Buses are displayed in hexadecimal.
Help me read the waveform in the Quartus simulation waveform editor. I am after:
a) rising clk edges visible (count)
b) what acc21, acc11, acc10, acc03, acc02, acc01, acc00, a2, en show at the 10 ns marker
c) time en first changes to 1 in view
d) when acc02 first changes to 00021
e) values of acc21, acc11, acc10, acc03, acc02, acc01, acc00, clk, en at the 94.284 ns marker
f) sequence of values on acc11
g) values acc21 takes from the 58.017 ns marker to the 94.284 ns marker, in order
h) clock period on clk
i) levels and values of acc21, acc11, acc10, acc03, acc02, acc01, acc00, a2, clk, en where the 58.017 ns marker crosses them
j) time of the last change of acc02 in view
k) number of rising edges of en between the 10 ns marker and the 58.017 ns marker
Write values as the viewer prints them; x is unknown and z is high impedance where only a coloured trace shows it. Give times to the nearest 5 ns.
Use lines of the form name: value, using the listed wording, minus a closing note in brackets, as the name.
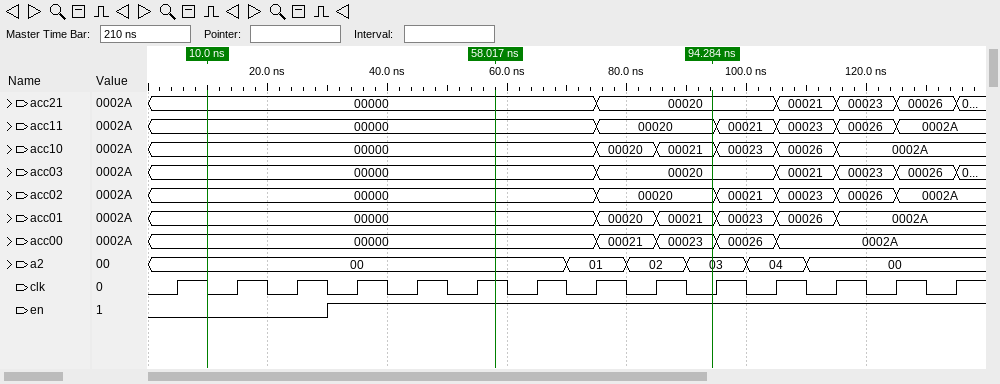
rising clk edges visible: 14
what acc21, acc11, acc10, acc03, acc02, acc01, acc00, a2, en show at the 10 ns marker: acc21=00000, acc11=00000, acc10=00000, acc03=00000, acc02=00000, acc01=00000, acc00=00000, a2=00, en=0
time en first changes to 1 in view: 30 ns
when acc02 first changes to 00021: 95 ns
values of acc21, acc11, acc10, acc03, acc02, acc01, acc00, clk, en at the 94.284 ns marker: acc21=00020, acc11=00020, acc10=00021, acc03=00020, acc02=00020, acc01=00021, acc00=00023, clk=0, en=1
sequence of values on acc11: 00000, 00020, 00021, 00023, 00026, 0002A
values acc21 takes from the 58.017 ns marker to the 94.284 ns marker, in order: 00000, 00020
clock period on clk: 10 ns
levels and values of acc21, acc11, acc10, acc03, acc02, acc01, acc00, a2, clk, en where the 58.017 ns marker crosses them: acc21=00000, acc11=00000, acc10=00000, acc03=00000, acc02=00000, acc01=00000, acc00=00000, a2=00, clk=1, en=1
time of the last change of acc02 in view: 125 ns
number of rising edges of en between the 10 ns marker and the 58.017 ns marker: 1
